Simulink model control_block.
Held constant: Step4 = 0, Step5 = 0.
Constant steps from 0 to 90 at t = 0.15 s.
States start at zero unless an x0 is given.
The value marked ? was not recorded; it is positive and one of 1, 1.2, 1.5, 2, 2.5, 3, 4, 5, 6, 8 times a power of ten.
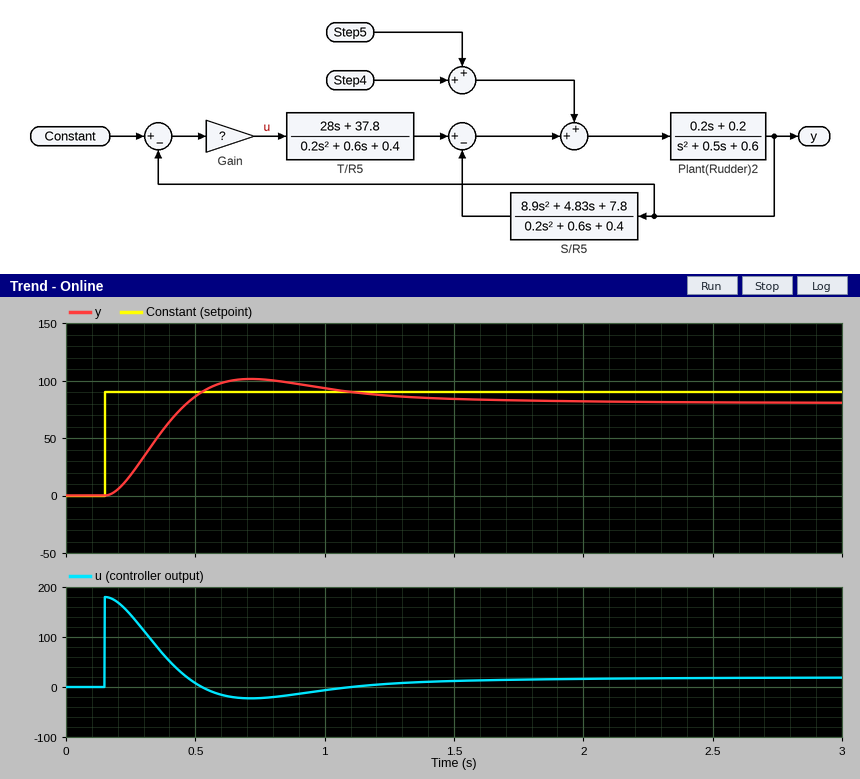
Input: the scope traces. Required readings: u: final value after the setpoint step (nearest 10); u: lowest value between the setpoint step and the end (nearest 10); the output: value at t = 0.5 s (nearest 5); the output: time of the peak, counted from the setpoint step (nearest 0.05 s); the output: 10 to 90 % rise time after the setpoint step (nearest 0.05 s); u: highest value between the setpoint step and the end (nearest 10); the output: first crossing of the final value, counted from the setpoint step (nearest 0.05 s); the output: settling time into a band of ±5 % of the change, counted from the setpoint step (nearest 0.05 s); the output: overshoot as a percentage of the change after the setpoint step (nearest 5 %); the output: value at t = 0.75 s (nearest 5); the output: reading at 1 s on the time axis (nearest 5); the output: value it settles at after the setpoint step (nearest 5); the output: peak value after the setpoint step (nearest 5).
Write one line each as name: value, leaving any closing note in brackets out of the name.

u: final value after the setpoint step: 20
u: lowest value between the setpoint step and the end: -20
the output: value at t = 0.5 s: 85
the output: time of the peak, counted from the setpoint step: 0.55 s
the output: 10 to 90 % rise time after the setpoint step: 0.20 s
u: highest value between the setpoint step and the end: 180
the output: first crossing of the final value, counted from the setpoint step: 0.30 s
the output: settling time into a band of ±5 % of the change, counted from the setpoint step: 1.30 s
the output: overshoot as a percentage of the change after the setpoint step: 25 %
the output: value at t = 0.75 s: 100
the output: reading at 1 s on the time axis: 95
the output: value it settles at after the setpoint step: 80
the output: peak value after the setpoint step: 100
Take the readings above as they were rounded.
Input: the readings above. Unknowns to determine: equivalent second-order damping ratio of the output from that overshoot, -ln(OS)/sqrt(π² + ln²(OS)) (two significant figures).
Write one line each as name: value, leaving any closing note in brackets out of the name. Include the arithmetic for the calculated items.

equivalent second-order damping ratio of the output from that overshoot, -ln(OS)/sqrt(π² + ln²(OS)): ln(0.25) = -1.386; 1.386 / sqrt(9.870 + 1.922) = 0.40
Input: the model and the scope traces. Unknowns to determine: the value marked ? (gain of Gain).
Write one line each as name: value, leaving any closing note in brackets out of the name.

the value marked ?: 2
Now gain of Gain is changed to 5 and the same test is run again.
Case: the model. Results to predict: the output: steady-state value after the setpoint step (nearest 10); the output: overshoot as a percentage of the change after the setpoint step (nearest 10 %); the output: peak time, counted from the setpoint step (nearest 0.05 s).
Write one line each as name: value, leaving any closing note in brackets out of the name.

the output: steady-state value after the setpoint step: 90
the output: overshoot as a percentage of the change after the setpoint step: 30 %
the output: peak time, counted from the setpoint step: 0.30 s
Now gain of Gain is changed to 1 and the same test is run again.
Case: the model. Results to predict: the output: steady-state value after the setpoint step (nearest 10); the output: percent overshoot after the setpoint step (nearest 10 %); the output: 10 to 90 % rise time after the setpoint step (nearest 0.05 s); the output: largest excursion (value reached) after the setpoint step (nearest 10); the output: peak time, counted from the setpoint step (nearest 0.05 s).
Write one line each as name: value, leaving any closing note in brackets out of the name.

the output: steady-state value after the setpoint step: 70
the output: percent overshoot after the setpoint step: 30 %
the output: 10 to 90 % rise time after the setpoint step: 0.35 s
the output: largest excursion (value reached) after the setpoint step: 90
the output: peak time, counted from the setpoint step: 0.95 s
